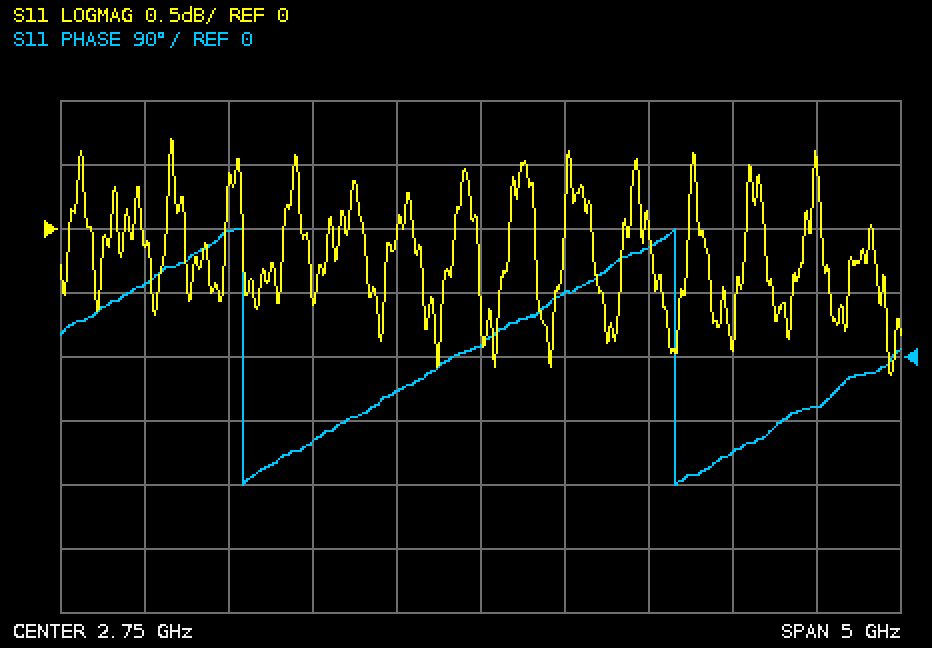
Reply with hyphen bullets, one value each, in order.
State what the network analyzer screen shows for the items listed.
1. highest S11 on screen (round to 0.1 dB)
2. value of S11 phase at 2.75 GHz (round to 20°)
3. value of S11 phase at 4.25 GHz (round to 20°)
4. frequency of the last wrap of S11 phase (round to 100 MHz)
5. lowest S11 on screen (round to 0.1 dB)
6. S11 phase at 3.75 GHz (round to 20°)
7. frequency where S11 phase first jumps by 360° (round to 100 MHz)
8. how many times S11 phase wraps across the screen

- 0.7 dB
- 20°
- -140°
- 3.9 GHz
- -1.1 dB
- 160°
- 1.3 GHz
- 2
